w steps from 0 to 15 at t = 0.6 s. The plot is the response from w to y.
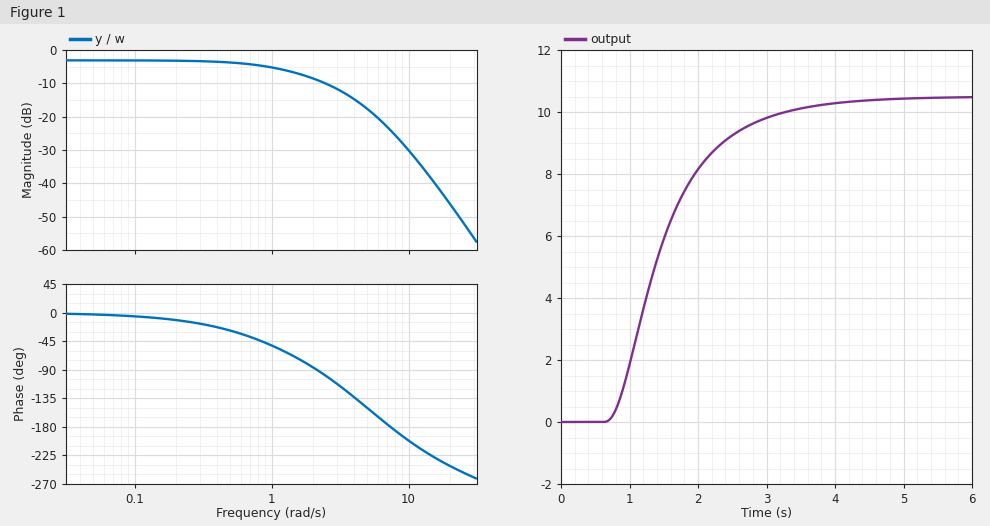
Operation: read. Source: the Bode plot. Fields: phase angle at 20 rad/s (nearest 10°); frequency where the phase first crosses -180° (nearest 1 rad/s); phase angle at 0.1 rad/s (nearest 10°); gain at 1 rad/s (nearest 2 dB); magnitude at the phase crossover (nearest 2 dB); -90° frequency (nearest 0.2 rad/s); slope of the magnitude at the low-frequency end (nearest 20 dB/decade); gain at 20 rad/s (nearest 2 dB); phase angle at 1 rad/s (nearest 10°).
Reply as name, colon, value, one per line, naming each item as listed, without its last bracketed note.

phase angle at 20 rad/s: -240°
frequency where the phase first crosses -180°: 7 rad/s
phase angle at 0.1 rad/s: -10°
gain at 1 rad/s: -6 dB
magnitude at the phase crossover: -24 dB
-90° frequency: 2.2 rad/s
slope of the magnitude at the low-frequency end: 0 dB/decade
gain at 20 rad/s: -46 dB
phase angle at 1 rad/s: -50°
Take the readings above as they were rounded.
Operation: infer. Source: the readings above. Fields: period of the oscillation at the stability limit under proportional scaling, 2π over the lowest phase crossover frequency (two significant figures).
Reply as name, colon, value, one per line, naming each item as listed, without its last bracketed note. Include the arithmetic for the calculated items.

period of the oscillation at the stability limit under proportional scaling, 2π over the lowest phase crossover frequency: 2π / 7 = 0.90 s
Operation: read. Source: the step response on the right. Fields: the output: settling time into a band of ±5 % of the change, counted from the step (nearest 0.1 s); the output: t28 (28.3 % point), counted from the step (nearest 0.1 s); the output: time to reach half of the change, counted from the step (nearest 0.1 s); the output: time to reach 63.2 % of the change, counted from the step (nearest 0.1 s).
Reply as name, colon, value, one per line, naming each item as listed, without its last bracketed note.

the output: settling time into a band of ±5 % of the change, counted from the step: 2.6 s
the output: t28 (28.3 % point), counted from the step: 0.5 s
the output: time to reach half of the change, counted from the step: 0.8 s
the output: time to reach 63.2 % of the change, counted from the step: 1.0 s
